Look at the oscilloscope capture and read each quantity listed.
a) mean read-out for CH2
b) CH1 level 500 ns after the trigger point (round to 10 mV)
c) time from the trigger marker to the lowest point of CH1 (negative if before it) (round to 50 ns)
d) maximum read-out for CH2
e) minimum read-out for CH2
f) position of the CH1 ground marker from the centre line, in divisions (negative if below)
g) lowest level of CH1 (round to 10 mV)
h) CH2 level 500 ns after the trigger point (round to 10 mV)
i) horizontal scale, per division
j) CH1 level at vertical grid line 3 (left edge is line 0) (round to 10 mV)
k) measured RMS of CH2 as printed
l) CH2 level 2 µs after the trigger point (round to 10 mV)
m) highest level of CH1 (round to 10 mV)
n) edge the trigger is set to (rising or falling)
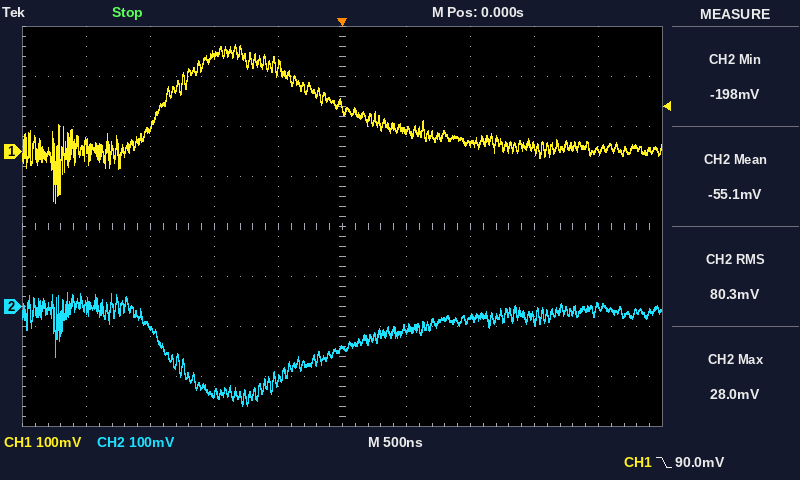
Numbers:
-55.1 mV
40 mV
-2.25 µs
28.0 mV
-198 mV
+1.5 div
-100 mV
-40 mV
500 ns
190 mV
80.3 mV
0 mV
210 mV
falling
